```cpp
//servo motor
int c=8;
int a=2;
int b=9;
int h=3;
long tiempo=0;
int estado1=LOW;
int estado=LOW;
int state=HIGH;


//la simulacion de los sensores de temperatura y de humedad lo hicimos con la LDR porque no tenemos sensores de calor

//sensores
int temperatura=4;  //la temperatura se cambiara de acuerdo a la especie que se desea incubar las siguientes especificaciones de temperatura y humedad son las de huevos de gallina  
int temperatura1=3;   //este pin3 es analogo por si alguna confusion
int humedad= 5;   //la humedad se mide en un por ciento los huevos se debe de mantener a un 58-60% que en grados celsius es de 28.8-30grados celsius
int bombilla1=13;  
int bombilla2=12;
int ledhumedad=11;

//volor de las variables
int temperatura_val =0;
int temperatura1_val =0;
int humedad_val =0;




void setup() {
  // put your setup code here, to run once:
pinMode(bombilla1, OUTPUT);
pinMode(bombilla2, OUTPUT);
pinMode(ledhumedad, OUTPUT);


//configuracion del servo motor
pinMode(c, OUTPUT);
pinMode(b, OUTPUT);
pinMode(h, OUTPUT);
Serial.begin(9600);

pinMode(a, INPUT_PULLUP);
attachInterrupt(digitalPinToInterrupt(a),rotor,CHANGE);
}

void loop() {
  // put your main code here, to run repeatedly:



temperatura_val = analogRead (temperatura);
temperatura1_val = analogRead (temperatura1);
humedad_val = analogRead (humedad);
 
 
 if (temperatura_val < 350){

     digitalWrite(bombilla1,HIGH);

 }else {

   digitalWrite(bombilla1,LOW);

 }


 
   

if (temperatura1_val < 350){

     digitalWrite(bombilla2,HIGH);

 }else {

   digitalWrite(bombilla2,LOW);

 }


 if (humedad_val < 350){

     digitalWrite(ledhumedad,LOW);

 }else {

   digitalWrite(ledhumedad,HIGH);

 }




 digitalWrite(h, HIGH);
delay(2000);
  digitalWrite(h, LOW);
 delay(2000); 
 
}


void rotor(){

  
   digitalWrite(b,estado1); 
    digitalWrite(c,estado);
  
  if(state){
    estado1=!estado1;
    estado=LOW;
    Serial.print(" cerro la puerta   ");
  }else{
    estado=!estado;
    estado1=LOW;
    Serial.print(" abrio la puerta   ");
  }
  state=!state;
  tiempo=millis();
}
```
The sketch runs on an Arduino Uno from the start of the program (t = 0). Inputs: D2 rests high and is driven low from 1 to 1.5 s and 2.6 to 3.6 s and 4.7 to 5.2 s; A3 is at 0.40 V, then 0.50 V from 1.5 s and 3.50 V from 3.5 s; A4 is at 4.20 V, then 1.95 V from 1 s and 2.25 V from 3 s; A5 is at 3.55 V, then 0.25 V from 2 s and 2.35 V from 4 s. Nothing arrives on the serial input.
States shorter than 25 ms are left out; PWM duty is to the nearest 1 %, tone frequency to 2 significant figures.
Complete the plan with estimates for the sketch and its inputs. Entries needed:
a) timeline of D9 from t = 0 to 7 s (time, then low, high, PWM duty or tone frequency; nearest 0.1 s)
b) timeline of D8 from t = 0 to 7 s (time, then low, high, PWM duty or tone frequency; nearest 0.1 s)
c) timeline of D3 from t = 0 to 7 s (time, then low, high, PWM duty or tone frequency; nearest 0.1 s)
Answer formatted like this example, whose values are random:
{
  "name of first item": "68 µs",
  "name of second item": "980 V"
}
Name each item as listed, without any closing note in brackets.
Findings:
{
  "timeline of D9 from t = 0 to 7 s": "0 s low; 1.5 s high; 2.6 s low; 3.6 s high; 4.7 s low; 5.2 s high",
  "timeline of D8 from t = 0 to 7 s": "0 s low; 2.6 s high; 3.6 s low; 4.7 s high; 5.2 s low",
  "timeline of D3 from t = 0 to 7 s": "0 s high; 2 s low; 4 s high; 6 s low"
}
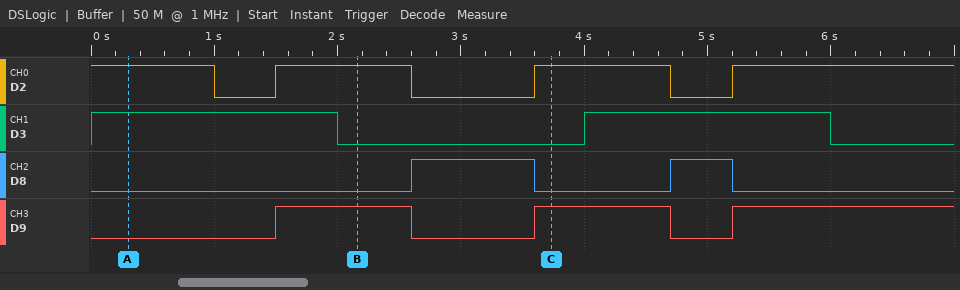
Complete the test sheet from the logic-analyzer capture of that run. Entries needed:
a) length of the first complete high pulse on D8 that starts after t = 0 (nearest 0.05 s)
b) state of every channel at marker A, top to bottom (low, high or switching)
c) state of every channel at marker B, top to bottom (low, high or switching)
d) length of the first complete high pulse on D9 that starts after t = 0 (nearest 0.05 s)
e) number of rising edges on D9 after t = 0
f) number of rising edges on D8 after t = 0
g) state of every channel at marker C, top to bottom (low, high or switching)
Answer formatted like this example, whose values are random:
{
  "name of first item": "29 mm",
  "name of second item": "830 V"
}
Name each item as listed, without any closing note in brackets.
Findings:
{
  "length of the first complete high pulse on D8 that starts after t = 0": "1.00 s",
  "state of every channel at marker A, top to bottom": "D2 high, D3 high, D8 low, D9 low",
  "state of every channel at marker B, top to bottom": "D2 high, D3 low, D8 low, D9 high",
  "length of the first complete high pulse on D9 that starts after t = 0": "1.10 s",
  "number of rising edges on D9 after t = 0": "3",
  "number of rising edges on D8 after t = 0": "2",
  "state of every channel at marker C, top to bottom": "D2 high, D3 low, D8 low, D9 high"
}
